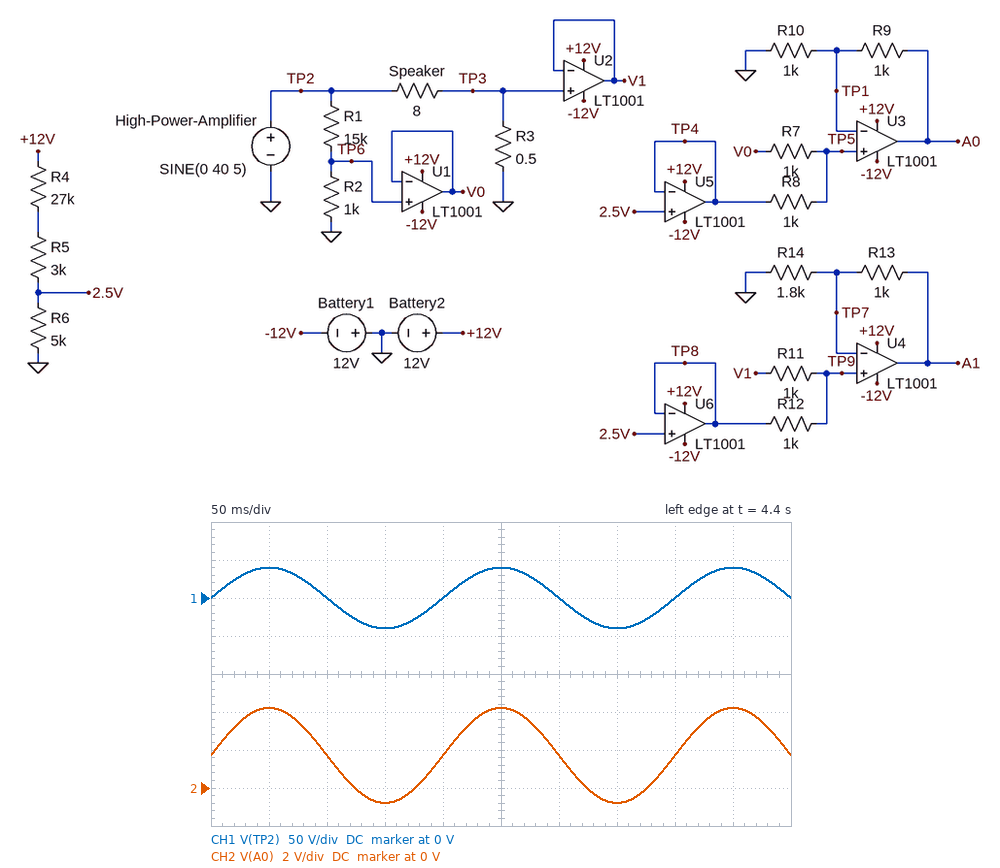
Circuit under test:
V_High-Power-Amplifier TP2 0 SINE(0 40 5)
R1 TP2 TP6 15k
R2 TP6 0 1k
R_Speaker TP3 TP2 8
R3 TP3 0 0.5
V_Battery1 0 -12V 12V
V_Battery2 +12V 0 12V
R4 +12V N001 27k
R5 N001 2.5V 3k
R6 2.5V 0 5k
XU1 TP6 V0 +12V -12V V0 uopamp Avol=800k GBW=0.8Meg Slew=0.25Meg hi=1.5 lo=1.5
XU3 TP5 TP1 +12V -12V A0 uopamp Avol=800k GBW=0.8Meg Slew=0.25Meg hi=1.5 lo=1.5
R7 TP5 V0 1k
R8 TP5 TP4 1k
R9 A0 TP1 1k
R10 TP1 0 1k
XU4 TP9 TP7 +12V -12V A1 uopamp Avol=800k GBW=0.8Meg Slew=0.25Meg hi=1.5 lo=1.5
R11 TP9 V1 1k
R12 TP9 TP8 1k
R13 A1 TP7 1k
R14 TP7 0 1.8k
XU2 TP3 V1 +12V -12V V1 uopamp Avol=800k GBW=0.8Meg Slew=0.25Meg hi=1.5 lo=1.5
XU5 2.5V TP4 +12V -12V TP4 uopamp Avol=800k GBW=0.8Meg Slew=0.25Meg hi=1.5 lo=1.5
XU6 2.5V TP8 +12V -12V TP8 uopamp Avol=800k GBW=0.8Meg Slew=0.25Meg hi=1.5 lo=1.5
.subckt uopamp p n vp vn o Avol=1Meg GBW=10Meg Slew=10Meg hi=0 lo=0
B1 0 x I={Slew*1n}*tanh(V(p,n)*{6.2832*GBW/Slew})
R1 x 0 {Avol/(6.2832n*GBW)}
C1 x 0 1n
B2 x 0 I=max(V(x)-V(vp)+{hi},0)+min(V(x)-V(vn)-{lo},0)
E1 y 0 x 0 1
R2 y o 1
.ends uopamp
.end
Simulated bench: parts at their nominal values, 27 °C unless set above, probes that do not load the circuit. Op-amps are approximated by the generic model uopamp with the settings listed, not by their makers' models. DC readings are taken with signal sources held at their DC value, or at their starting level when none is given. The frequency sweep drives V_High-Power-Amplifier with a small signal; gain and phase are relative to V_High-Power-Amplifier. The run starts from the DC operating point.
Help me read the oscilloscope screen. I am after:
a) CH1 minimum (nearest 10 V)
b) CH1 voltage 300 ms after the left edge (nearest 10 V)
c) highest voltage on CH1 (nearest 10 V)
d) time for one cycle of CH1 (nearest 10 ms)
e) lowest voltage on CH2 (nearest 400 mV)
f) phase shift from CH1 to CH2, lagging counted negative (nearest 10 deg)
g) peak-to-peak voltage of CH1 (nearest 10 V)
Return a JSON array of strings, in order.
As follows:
["-40 V", "0 V", "40 V", "200 ms", "-800 mV", "0 deg", "80 V"]
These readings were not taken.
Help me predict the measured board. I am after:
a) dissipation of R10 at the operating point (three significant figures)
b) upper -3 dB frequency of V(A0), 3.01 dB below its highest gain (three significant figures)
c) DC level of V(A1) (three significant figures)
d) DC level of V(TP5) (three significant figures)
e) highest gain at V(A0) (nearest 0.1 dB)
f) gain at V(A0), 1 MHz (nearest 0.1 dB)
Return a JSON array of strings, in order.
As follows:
["735 µW", "335 kHz", "1.33 V", "857 mV", "-24.1 dB", "-36.8 dB"]
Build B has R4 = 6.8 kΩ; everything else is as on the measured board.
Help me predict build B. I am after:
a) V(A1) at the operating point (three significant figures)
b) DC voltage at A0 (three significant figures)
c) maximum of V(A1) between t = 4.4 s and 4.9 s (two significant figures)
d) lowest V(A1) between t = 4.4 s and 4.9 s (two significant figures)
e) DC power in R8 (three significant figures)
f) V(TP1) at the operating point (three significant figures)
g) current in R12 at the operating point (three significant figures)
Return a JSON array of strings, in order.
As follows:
["3.15 V", "4.05 V", "5.0 V", "1.3 V", "4.11 mW", "2.03 V", "2.03 mA"]
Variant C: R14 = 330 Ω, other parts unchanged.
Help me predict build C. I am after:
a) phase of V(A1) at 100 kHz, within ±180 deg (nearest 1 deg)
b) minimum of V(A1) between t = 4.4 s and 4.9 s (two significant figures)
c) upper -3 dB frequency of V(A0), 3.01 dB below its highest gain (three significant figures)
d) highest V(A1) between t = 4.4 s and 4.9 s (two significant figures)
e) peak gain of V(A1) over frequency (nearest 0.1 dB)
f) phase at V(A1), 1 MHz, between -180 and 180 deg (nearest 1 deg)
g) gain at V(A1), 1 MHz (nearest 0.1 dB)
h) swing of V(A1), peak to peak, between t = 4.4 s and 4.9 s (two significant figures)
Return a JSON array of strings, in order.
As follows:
["-34 deg", "-1.3 V", "335 kHz", "8.2 V", "-18.5 dB", "-130 deg", "-36.8 dB", "9.5 V"]
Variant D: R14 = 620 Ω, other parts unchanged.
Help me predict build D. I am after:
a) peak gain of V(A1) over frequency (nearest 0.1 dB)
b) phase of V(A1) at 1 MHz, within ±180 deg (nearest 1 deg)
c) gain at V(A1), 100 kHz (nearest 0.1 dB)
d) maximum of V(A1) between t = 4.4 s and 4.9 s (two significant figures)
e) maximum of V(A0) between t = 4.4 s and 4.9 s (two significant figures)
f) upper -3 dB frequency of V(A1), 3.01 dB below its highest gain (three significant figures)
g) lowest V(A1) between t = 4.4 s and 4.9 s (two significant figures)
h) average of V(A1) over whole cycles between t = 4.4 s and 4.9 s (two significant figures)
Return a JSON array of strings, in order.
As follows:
["-22.3 dB", "-124 deg", "-22.8 dB", "5.3 V", "4.2 V", "272 kHz", "-830 mV", "2.2 V"]
